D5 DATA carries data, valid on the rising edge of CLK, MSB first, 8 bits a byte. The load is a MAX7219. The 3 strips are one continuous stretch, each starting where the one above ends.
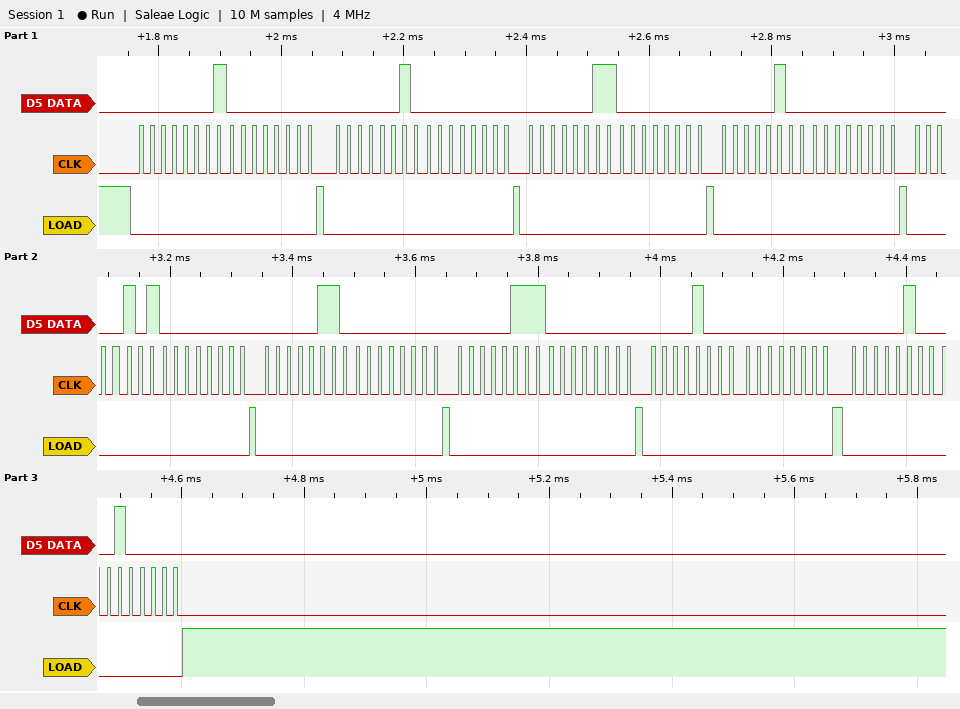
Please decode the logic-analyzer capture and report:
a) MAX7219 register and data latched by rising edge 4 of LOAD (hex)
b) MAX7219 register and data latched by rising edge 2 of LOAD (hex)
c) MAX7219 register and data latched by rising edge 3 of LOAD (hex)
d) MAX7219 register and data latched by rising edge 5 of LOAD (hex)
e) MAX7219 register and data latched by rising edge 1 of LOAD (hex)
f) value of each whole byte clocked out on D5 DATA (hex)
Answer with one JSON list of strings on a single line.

["register 0x4, data 0x00", "register 0x2, data 0x00", "register 0x3, data 0x00", "register 0x5, data 0x00", "register 0x1, data 0x00", "0x01 0x00 0x02 0x00 0x03 0x00 0x04 0x00 0x05 0x00 0x06 0x00 0x07 0x00 0x08 0x00 0x04 0x20"]
